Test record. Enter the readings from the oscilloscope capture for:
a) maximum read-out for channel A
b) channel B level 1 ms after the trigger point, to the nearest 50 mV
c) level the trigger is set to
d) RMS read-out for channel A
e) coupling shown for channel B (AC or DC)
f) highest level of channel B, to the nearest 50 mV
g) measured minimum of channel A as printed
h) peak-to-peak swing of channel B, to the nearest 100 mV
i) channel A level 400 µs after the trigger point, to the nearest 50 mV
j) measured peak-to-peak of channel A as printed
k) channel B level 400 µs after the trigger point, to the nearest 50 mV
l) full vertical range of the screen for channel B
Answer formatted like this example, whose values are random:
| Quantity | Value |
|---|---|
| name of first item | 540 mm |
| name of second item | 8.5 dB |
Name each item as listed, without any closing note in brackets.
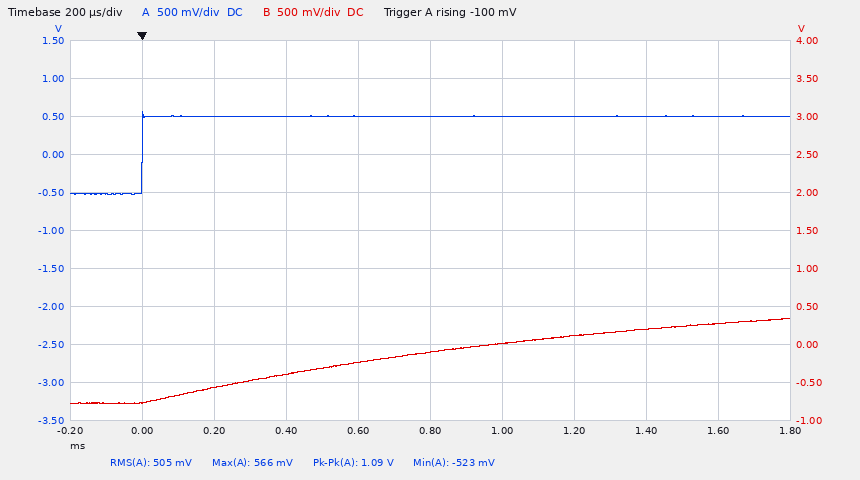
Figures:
| Quantity | Value |
|---|---|
| maximum read-out for channel A | 566 mV |
| channel B level 1 ms after the trigger point, to the nearest 50 mV | 0 mV |
| level the trigger is set to | -100 mV |
| RMS read-out for channel A | 505 mV |
| coupling shown for channel B | DC |
| highest level of channel B, to the nearest 50 mV | 350 mV |
| measured minimum of channel A as printed | -523 mV |
| peak-to-peak swing of channel B, to the nearest 100 mV | 1.10 V |
| channel A level 400 µs after the trigger point, to the nearest 50 mV | 500 mV |
| measured peak-to-peak of channel A as printed | 1.09 V |
| channel B level 400 µs after the trigger point, to the nearest 50 mV | -400 mV |
| full vertical range of the screen for channel B | 5 V |
